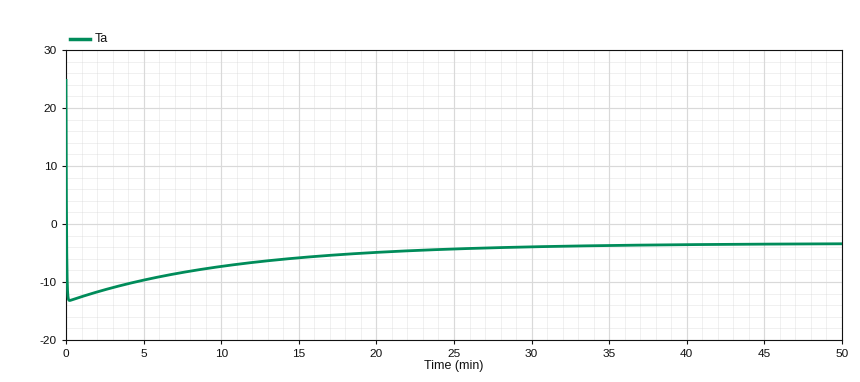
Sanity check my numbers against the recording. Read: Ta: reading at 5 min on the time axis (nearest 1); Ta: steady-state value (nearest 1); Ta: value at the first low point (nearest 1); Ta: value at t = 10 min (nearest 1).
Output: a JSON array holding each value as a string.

["-10", "-3", "-13", "-7"]
